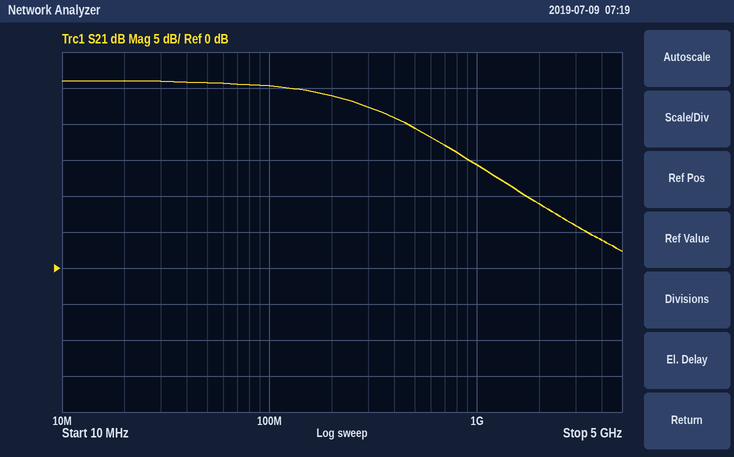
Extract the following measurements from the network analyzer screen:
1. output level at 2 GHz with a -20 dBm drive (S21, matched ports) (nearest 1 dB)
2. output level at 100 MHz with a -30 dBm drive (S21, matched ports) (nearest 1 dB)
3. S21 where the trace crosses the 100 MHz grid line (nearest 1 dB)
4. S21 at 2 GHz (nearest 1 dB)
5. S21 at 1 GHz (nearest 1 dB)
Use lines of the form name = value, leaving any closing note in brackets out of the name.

output level at 2 GHz with a -20 dBm drive (S21, matched ports) = -11 dBm
output level at 100 MHz with a -30 dBm drive (S21, matched ports) = -5 dBm
S21 where the trace crosses the 100 MHz grid line = 25 dB
S21 at 2 GHz = 9 dB
S21 at 1 GHz = 14 dB
